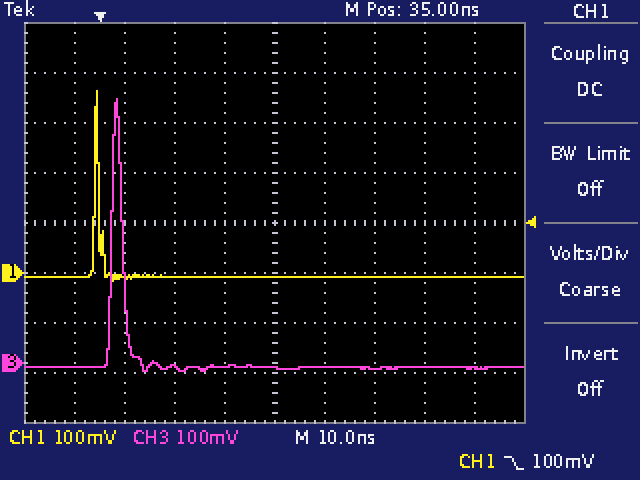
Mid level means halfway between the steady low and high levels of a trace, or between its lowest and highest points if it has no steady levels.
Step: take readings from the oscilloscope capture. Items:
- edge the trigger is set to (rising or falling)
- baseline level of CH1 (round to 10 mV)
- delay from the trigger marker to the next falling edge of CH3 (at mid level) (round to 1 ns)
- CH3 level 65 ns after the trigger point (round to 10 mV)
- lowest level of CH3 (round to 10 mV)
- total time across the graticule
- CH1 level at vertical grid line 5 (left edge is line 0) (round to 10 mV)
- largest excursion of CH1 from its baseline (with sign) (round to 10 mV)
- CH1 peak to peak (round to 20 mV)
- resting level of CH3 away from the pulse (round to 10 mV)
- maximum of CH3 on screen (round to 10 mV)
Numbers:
falling
-10 mV
5 ns
-10 mV
-20 mV
100 ns
-10 mV
+370 mV
380 mV
-10 mV
530 mV
